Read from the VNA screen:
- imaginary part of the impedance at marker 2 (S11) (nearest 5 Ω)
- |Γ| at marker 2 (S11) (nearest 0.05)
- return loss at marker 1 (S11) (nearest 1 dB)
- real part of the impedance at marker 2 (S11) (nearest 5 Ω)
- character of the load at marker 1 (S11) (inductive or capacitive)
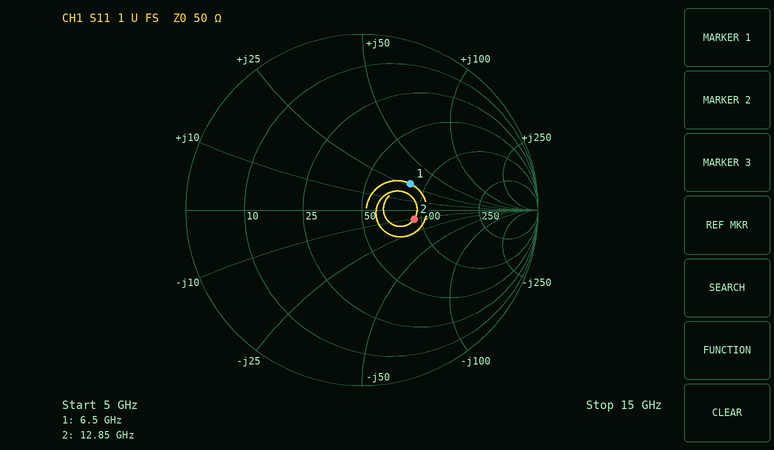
-10 Ω
0.30
10 dB
90 Ω
inductive
